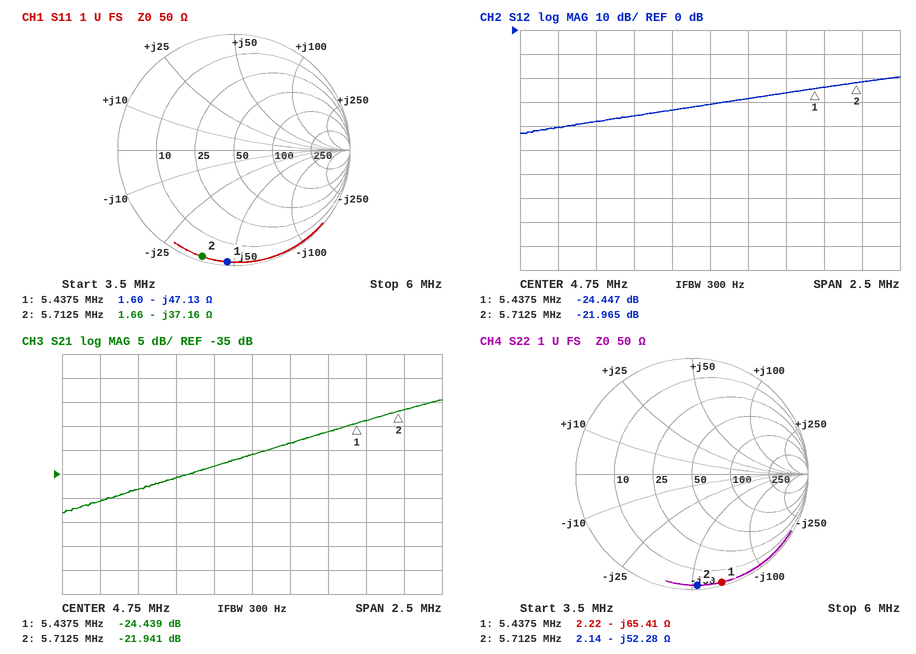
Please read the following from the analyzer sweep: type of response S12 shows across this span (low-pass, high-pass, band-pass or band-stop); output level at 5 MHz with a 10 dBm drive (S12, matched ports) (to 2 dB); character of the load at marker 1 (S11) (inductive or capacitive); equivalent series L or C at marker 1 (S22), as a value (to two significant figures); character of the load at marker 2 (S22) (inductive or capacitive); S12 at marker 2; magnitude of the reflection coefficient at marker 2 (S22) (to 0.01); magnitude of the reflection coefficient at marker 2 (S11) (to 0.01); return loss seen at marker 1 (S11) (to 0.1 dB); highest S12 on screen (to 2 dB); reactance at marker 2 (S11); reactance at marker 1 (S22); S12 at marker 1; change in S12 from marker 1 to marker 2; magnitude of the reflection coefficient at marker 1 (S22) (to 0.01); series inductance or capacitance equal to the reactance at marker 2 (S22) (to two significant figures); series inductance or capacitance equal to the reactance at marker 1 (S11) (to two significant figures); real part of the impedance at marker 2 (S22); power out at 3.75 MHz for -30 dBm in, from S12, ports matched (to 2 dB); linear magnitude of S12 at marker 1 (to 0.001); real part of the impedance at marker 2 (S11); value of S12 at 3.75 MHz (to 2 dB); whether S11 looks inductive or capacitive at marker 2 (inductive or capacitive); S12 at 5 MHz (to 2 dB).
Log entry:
high-pass
-18 dBm
capacitive
450 pF
capacitive
-21.965 dB
0.96
0.96
0.3 dB
-20 dB
-37.16 Ω
-65.41 Ω
-24.447 dB
2.482 dB
0.97
530 pF
620 pF
2.14 Ω
-70 dBm
0.060
1.66 Ω
-40 dB
capacitive
-28 dB
